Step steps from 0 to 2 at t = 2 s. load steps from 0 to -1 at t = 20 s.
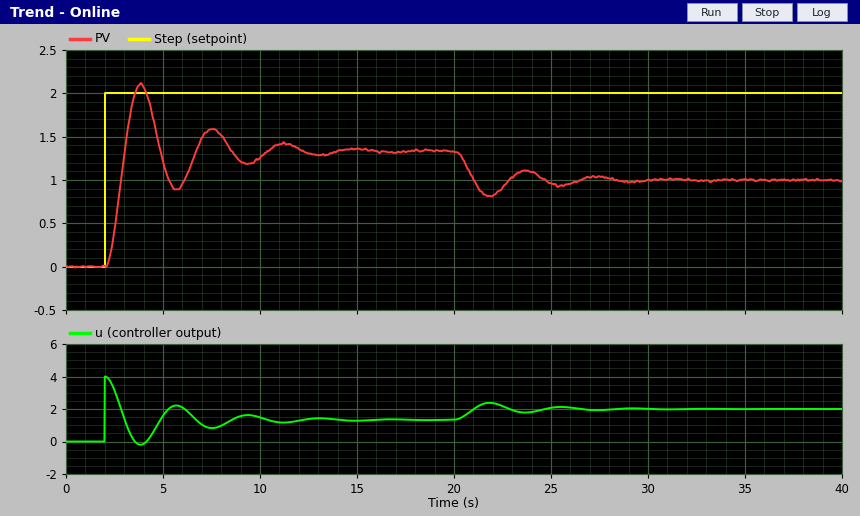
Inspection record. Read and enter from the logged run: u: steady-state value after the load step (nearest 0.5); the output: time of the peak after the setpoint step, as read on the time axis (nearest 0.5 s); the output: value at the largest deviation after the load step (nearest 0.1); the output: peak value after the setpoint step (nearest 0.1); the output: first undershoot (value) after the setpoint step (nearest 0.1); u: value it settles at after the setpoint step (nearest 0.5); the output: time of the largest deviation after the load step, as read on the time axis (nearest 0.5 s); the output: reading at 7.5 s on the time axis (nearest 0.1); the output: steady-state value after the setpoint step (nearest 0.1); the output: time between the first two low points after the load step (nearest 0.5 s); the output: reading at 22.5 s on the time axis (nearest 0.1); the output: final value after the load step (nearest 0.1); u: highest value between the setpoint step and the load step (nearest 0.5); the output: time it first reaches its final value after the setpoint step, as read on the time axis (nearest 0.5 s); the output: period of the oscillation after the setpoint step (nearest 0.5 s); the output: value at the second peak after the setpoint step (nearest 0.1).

2.0
4.0 s
0.8
2.1
0.9
1.5
22.0 s
1.6
1.3
3.5 s
0.9
1.0
4.0
3.0 s
3.5 s
1.6
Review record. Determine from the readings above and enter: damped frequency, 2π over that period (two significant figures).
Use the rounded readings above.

1.8 rad/s
